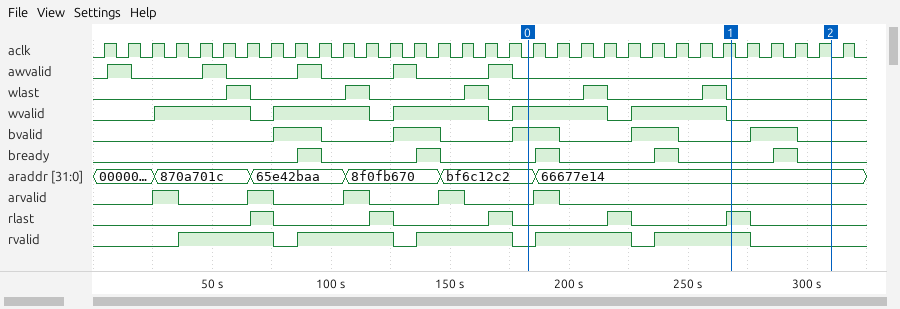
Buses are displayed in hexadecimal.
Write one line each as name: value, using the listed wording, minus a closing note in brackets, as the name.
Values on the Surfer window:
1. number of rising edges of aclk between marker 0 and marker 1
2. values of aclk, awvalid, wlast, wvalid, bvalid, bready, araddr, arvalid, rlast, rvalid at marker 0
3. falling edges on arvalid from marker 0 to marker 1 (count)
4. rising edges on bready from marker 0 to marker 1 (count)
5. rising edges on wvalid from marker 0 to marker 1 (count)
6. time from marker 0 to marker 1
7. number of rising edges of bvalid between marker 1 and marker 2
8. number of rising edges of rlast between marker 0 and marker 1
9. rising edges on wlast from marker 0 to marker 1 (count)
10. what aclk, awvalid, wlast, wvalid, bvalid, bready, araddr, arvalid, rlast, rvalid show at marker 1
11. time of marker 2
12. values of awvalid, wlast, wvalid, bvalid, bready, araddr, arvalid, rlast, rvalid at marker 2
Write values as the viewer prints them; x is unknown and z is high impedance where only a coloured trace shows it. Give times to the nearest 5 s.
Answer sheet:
number of rising edges of aclk between marker 0 and marker 1: 9
values of aclk, awvalid, wlast, wvalid, bvalid, bready, araddr, arvalid, rlast, rvalid at marker 0: aclk=0, awvalid=0, wlast=0, wvalid=1, bvalid=1, bready=0, araddr=bf6c12c2, arvalid=0, rlast=0, rvalid=0
falling edges on arvalid from marker 0 to marker 1: 1
rising edges on bready from marker 0 to marker 1: 2
rising edges on wvalid from marker 0 to marker 1: 1
time from marker 0 to marker 1: 85 s
number of rising edges of bvalid between marker 1 and marker 2: 1
number of rising edges of rlast between marker 0 and marker 1: 2
rising edges on wlast from marker 0 to marker 1: 2
what aclk, awvalid, wlast, wvalid, bvalid, bready, araddr, arvalid, rlast, rvalid show at marker 1: aclk=1, awvalid=0, wlast=0, wvalid=0, bvalid=0, bready=0, araddr=66677e14, arvalid=0, rlast=1, rvalid=1
time of marker 2: 310 s
values of awvalid, wlast, wvalid, bvalid, bready, araddr, arvalid, rlast, rvalid at marker 2: awvalid=0, wlast=0, wvalid=0, bvalid=0, bready=0, araddr=66677e14, arvalid=0, rlast=0, rvalid=0
